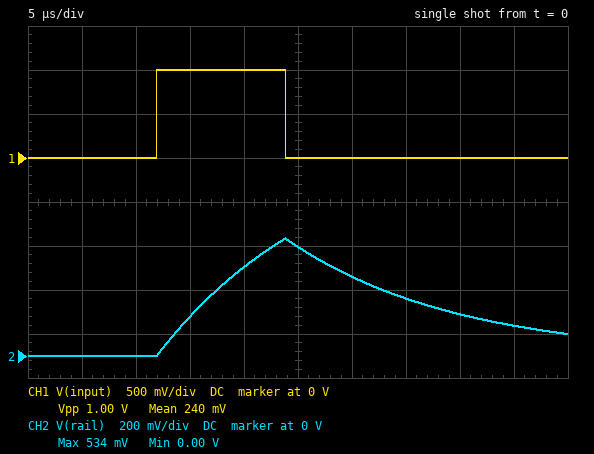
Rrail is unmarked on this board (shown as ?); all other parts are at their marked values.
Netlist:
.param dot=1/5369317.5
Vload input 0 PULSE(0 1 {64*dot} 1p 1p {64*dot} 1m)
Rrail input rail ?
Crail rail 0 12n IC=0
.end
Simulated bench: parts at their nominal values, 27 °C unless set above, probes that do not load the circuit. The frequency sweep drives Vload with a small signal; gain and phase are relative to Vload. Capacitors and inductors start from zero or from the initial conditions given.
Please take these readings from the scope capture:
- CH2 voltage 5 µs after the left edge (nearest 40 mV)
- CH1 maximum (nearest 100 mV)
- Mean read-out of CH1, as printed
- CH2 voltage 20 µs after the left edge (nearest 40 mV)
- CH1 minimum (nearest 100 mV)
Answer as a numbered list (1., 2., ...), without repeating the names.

1. 0 V
2. 1.0 V
3. 240 mV
4. 400 mV
5. 0 V
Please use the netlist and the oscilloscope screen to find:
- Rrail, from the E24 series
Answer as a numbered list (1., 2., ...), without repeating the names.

1. 1.3 kΩ
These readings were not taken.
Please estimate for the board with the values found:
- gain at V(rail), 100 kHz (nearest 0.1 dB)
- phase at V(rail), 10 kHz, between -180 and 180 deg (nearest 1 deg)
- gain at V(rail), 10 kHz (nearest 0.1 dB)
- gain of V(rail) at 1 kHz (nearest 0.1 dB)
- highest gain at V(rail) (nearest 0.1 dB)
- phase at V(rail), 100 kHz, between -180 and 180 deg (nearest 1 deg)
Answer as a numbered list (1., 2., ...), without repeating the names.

1. -19.9 dB
2. -44 deg
3. -2.9 dB
4. 0 dB
5. 0 dB
6. -84 deg
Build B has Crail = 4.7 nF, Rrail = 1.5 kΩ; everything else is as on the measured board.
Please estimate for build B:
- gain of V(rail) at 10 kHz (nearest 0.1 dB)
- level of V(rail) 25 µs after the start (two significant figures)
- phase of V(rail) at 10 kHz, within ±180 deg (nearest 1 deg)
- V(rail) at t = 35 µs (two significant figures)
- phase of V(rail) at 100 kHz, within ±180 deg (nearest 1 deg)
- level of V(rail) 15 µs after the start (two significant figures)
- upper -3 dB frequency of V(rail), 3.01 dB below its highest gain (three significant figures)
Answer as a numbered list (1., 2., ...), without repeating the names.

1. -0.8 dB
2. 690 mV
3. -24 deg
4. 170 mV
5. -77 deg
6. 350 mV
7. 22.6 kHz
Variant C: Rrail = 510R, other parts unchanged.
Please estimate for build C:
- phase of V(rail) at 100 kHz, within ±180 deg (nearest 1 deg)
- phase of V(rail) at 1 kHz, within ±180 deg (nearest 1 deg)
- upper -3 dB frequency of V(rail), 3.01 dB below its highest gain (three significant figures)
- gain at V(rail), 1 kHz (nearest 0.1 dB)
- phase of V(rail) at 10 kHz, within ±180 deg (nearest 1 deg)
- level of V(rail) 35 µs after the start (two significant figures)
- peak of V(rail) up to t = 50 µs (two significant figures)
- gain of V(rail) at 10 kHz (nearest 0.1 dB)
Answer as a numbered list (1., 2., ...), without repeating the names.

1. -75 deg
2. -2 deg
3. 26.0 kHz
4. 0 dB
5. -21 deg
6. 140 mV
7. 860 mV
8. -0.6 dB
